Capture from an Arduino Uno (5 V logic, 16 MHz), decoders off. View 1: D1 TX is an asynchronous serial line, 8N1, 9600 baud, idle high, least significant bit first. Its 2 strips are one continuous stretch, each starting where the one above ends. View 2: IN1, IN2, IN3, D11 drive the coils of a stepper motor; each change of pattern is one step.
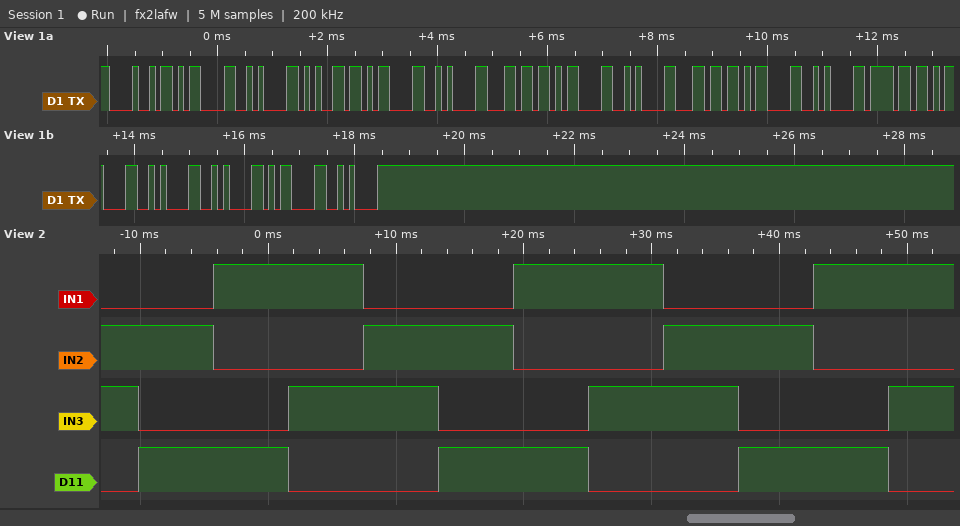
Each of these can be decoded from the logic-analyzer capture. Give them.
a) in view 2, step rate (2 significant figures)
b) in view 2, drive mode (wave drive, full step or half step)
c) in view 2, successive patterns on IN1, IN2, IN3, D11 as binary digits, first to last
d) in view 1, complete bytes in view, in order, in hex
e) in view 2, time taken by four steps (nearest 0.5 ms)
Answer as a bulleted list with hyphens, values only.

- 170 steps/s
- full step
- 0110 0101 1001 1010 0110 0101 1001 1010 0110 0101 1001 1010
- 48 0D 0A 65 0D 0A 6C 0D 0A 6C 0D 0A 6F 0D 0A 0A 0D 0A
- 23.5 ms
